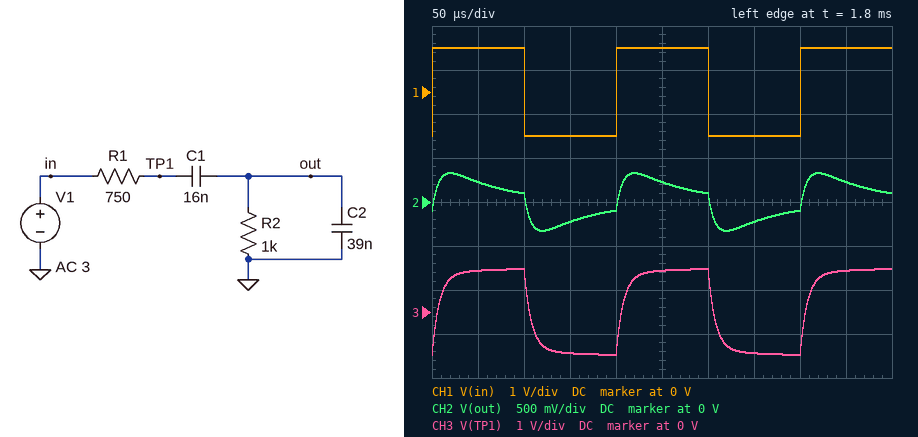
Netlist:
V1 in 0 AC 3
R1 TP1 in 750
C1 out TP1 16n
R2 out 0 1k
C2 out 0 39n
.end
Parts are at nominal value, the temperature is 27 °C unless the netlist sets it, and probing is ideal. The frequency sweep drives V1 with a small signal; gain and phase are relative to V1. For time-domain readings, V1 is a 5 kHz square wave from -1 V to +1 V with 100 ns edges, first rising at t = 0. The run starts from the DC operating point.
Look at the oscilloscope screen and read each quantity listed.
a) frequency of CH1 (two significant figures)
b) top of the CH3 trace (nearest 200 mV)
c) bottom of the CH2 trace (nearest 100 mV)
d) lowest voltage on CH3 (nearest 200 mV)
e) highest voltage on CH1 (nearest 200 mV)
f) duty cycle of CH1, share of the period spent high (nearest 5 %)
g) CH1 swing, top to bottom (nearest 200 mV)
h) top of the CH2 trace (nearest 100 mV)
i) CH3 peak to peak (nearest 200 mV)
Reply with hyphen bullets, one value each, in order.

- 5.0 kHz
- 1.0 V
- -300 mV
- -1.0 V
- 1.0 V
- 50 %
- 2.0 V
- 300 mV
- 2.0 V
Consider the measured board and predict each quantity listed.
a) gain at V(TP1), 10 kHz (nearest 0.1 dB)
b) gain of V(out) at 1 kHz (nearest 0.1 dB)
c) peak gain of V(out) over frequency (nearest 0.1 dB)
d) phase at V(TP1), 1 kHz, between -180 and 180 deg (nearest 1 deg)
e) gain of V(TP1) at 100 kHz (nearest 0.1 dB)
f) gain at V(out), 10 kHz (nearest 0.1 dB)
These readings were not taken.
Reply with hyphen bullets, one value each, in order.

- -1.5 dB
- -20.5 dB
- -12.4 dB
- -4 deg
- -14.7 dB
- -12.6 dB
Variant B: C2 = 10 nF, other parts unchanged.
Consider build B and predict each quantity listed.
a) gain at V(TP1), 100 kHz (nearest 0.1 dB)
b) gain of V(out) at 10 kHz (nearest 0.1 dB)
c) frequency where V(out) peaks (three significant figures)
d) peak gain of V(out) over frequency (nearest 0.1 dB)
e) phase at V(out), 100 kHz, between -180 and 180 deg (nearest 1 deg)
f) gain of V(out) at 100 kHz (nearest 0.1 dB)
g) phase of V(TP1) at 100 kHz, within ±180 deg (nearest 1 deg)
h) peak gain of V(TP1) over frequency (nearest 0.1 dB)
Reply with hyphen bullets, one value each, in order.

- -10.1 dB
- -7.7 dB
- 14.5 kHz
- -7.5 dB
- -63 deg
- -14.3 dB
- -66 deg
- 0 dB
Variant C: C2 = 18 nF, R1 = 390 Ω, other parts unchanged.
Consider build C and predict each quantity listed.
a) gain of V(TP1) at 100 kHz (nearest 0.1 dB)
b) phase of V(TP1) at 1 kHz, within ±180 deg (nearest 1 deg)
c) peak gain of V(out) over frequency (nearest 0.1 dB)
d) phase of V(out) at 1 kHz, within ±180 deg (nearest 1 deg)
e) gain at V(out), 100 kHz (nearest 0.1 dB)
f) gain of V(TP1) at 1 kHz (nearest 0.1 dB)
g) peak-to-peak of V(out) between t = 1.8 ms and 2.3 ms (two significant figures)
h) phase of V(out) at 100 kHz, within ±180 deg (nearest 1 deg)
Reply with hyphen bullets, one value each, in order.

- -7.4 dB
- -2 deg
- -8.0 dB
- 76 deg
- -14.0 dB
- 0 dB
- 1.3 V
- -60 deg
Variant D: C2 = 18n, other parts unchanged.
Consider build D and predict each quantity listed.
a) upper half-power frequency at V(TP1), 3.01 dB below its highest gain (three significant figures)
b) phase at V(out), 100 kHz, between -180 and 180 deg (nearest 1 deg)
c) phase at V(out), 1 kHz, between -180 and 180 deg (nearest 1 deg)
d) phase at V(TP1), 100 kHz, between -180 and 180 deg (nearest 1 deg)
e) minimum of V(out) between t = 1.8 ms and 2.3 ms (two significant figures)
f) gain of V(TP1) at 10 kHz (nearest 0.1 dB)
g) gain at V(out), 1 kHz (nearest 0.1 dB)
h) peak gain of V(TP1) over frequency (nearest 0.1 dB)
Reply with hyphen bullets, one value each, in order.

- 19.4 kHz
- -71 deg
- 74 deg
- -74 deg
- -530 mV
- -1.8 dB
- -20.2 dB
- 0 dB
